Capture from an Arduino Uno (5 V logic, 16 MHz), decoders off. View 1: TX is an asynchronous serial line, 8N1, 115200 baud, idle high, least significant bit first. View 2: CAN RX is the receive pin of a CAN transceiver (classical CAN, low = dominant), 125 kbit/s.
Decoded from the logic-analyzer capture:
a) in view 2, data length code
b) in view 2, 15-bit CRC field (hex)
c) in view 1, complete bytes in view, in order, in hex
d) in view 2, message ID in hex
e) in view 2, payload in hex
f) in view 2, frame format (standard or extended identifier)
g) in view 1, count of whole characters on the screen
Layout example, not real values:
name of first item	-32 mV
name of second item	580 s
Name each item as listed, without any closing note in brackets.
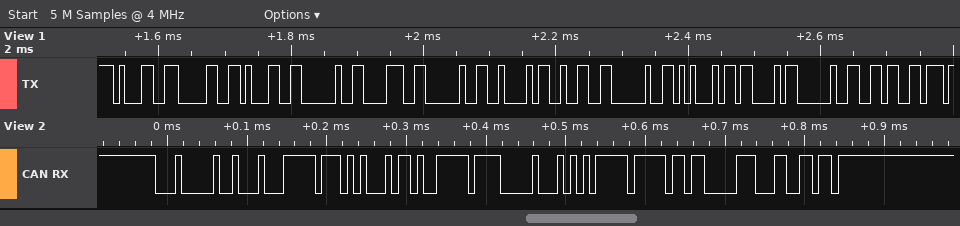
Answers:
in view 2, data length code	8
in view 2, 15-bit CRC field	0x18CD
in view 1, complete bytes in view, in order, in hex	31 30 31 20 38 20 42 32 20 45 43 20 36
in view 2, message ID in hex	0x101
in view 2, payload in hex	FF 51 69 FF 00 AB FF D8
in view 2, frame format	standard
in view 1, count of whole characters on the screen	13
